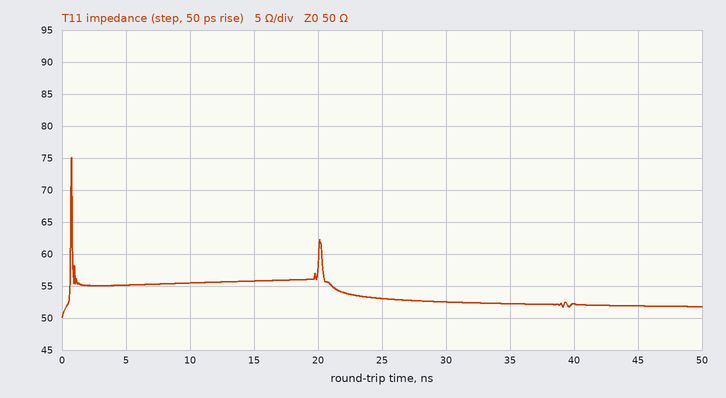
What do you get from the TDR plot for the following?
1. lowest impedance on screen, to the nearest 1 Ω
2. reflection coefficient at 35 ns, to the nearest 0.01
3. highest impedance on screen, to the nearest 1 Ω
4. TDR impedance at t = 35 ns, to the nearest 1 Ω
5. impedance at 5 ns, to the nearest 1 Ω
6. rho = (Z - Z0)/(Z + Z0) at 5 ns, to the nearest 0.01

50 Ω
+0.02
75 Ω
52 Ω
55 Ω
+0.05
